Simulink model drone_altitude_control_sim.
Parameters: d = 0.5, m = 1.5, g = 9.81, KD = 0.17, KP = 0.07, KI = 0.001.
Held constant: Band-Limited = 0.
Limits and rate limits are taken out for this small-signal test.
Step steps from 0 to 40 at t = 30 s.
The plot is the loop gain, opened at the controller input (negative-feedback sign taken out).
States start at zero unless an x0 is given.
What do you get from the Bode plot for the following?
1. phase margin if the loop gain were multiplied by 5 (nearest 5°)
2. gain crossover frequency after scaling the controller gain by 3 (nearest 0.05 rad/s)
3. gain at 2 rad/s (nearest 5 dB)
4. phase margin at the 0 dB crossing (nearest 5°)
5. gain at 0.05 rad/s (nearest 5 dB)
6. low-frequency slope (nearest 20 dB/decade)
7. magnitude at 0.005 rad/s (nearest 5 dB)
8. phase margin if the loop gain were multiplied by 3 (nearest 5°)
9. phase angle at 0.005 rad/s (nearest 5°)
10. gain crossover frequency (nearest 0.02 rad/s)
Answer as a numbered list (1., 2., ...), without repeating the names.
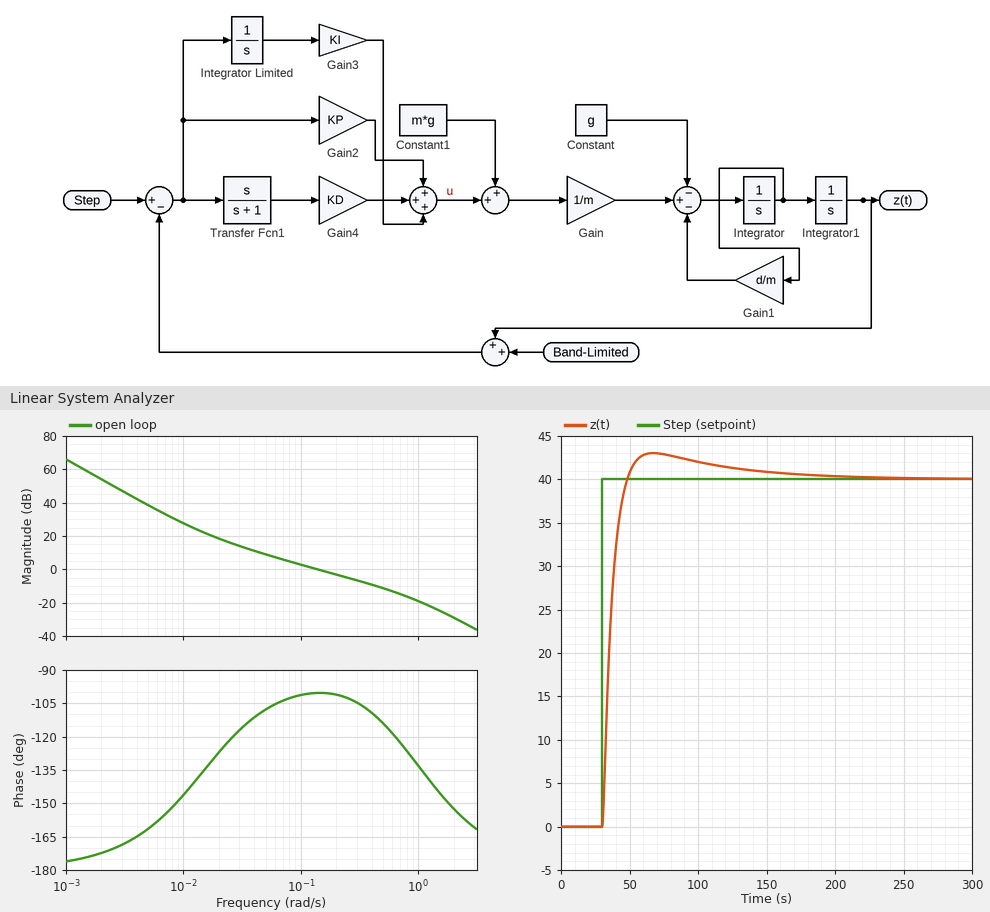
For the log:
1. 60°
2. 0.40 rad/s
3. -30 dB
4. 80°
5. 10 dB
6. -40 dB/decade
7. 40 dB
8. 70°
9. -160°
10. 0.14 rad/s
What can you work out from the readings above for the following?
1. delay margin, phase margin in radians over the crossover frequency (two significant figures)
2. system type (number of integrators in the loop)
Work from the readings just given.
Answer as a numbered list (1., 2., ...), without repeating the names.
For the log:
1. 10.0 s
2. 2
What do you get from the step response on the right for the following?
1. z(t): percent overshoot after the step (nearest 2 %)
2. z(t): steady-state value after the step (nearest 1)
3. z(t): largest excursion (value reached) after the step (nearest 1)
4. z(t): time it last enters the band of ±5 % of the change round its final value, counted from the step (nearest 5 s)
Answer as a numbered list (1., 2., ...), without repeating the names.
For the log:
1. 8 %
2. 40
3. 43
4. 70 s
